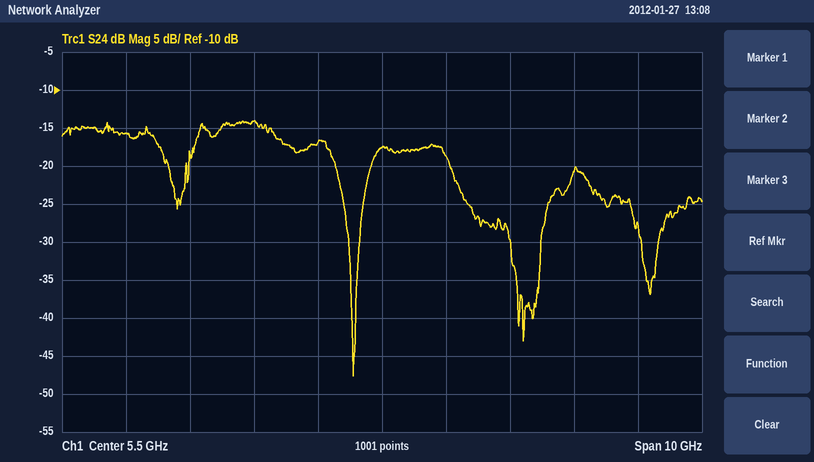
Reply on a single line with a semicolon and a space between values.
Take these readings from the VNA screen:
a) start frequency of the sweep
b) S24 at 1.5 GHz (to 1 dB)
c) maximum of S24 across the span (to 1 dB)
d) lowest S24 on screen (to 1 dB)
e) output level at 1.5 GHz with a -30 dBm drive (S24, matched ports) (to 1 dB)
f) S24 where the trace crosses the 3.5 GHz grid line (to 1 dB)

500 MHz; -16 dB; -14 dB; -48 dB; -46 dBm; -14 dB
